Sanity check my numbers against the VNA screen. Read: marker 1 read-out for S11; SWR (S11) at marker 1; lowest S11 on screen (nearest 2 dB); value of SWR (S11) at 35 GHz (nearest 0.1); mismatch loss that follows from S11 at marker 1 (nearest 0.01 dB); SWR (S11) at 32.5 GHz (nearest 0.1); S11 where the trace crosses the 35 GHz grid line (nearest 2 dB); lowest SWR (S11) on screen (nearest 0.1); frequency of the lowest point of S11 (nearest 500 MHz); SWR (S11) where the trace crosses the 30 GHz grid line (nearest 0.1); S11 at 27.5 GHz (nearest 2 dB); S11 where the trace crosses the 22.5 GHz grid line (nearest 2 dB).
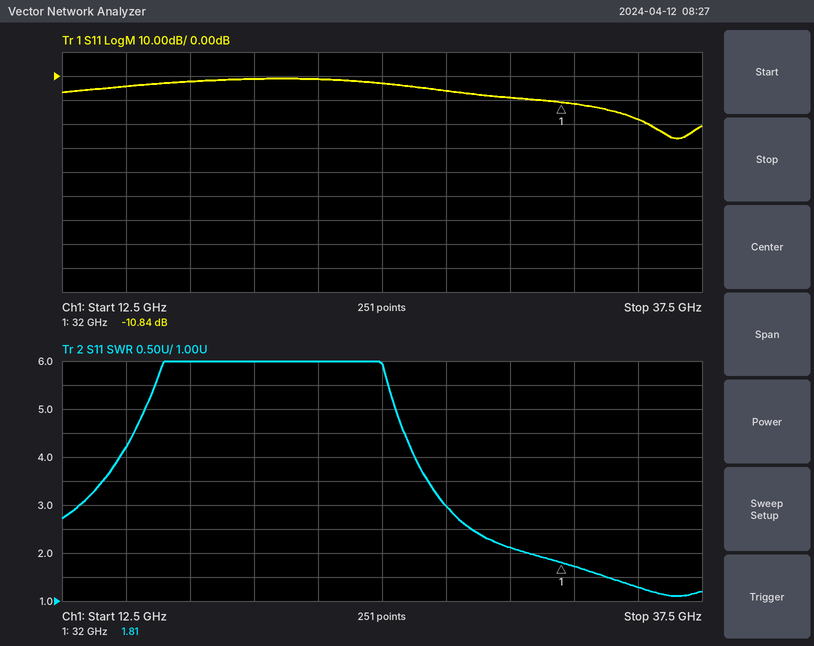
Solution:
-10.84 dB
1.81
-26 dB
1.3
0.37 dB
1.7
-18 dB
1.1
36.5 GHz
2.1
-6 dB
-2 dB
